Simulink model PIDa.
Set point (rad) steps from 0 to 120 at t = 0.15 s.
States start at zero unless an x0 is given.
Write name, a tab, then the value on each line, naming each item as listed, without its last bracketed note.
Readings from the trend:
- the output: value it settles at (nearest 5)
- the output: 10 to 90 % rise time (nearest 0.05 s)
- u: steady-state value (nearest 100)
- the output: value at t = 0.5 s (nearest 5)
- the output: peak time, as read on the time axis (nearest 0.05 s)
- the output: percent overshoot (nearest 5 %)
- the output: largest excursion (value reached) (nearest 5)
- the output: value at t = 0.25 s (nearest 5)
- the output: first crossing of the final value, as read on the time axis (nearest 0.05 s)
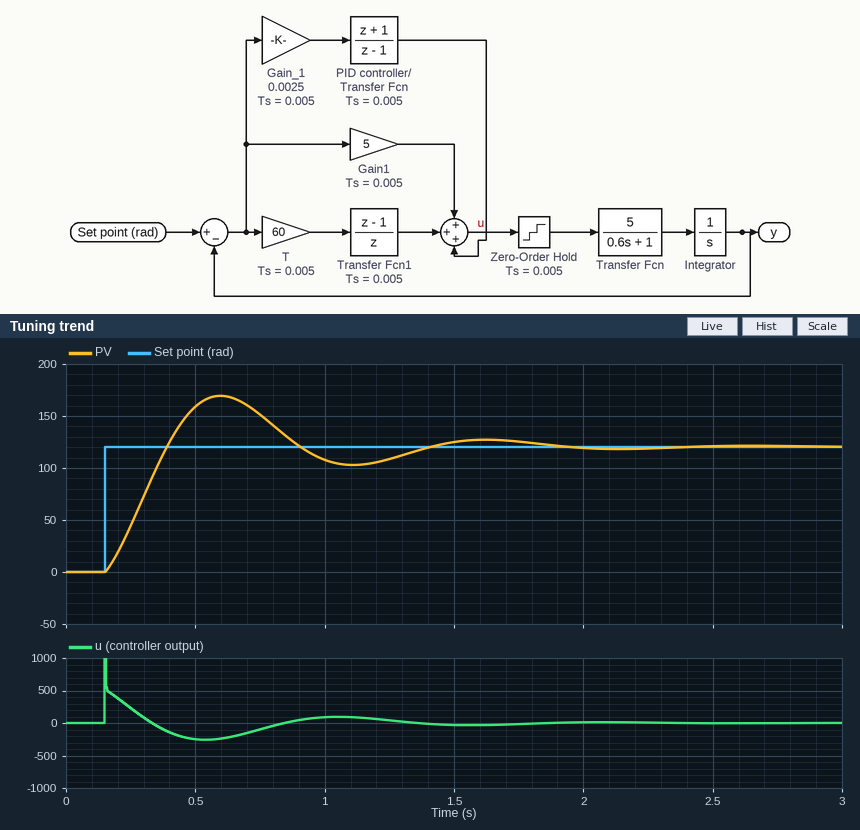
the output: value it settles at	120
the output: 10 to 90 % rise time	0.20 s
u: steady-state value	0
the output: value at t = 0.5 s	160
the output: peak time, as read on the time axis	0.60 s
the output: percent overshoot	40 %
the output: largest excursion (value reached)	170
the output: value at t = 0.25 s	45
the output: first crossing of the final value, as read on the time axis	0.40 s
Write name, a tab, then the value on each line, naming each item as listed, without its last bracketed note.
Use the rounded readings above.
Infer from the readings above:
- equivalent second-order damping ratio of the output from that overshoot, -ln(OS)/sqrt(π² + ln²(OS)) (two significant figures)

equivalent second-order damping ratio of the output from that overshoot, -ln(OS)/sqrt(π² + ln²(OS))	0.28
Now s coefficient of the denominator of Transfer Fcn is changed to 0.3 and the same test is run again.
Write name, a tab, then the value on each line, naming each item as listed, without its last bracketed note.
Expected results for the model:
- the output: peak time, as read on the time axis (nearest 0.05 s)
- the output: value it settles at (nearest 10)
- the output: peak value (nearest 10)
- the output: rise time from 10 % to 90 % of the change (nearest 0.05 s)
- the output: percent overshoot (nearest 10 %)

the output: peak time, as read on the time axis	0.45 s
the output: value it settles at	120
the output: peak value	150
the output: rise time from 10 % to 90 % of the change	0.15 s
the output: percent overshoot	30 %
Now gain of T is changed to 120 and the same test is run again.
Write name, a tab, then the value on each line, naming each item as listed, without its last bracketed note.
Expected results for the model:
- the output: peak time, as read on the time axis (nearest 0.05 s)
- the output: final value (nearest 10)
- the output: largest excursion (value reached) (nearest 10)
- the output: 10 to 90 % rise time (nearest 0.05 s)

the output: peak time, as read on the time axis	0.55 s
the output: final value	120
the output: largest excursion (value reached)	150
the output: 10 to 90 % rise time	0.15 s
